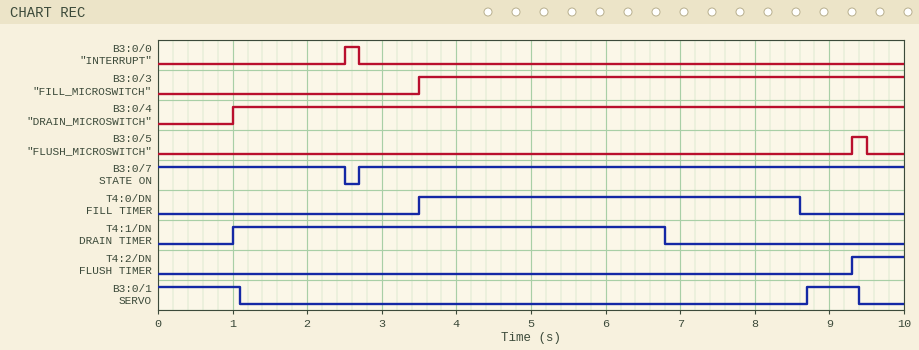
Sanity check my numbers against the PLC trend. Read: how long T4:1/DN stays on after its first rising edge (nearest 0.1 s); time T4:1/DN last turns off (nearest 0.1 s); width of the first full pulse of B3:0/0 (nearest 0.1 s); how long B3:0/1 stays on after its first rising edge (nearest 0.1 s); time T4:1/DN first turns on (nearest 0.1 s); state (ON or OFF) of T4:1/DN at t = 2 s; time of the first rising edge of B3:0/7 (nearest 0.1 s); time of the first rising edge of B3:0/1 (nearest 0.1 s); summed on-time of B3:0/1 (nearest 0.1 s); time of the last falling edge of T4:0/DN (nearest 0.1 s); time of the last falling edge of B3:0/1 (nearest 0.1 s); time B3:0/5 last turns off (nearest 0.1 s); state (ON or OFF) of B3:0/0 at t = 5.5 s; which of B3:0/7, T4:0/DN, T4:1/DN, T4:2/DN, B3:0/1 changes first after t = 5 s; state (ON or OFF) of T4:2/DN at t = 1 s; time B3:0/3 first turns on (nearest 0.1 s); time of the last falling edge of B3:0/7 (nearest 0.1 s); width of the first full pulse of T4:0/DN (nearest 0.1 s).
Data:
5.8 s
6.8 s
0.2 s
0.7 s
1.0 s
ON
2.7 s
8.7 s
1.8 s
8.6 s
9.4 s
9.5 s
OFF
T4:1/DN
OFF
3.5 s
2.5 s
5.1 s
